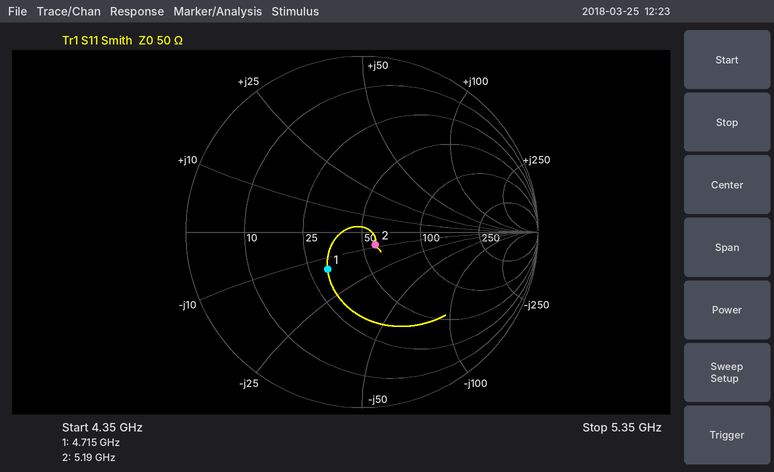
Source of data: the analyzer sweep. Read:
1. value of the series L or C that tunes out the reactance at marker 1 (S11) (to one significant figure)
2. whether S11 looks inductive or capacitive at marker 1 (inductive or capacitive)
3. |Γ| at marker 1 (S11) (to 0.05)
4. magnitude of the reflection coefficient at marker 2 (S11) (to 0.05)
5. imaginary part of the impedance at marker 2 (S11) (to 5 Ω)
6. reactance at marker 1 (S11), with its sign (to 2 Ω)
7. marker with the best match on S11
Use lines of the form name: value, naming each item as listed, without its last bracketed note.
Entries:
value of the series L or C that tunes out the reactance at marker 1 (S11): 500 pH
whether S11 looks inductive or capacitive at marker 1: capacitive
|Γ| at marker 1 (S11): 0.30
magnitude of the reflection coefficient at marker 2 (S11): 0.10
imaginary part of the impedance at marker 2 (S11): -10 Ω
reactance at marker 1 (S11), with its sign: -14 Ω
marker with the best match on S11: marker 2
